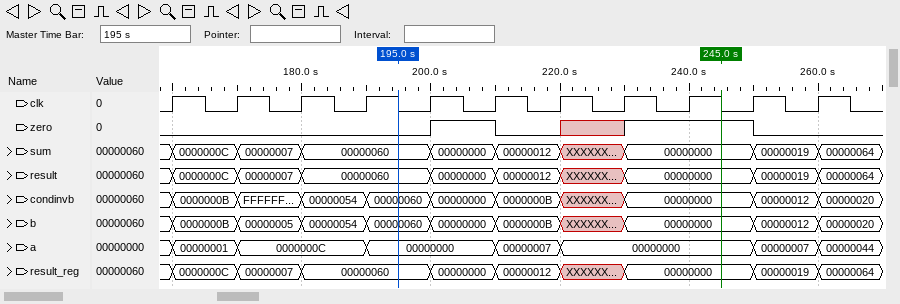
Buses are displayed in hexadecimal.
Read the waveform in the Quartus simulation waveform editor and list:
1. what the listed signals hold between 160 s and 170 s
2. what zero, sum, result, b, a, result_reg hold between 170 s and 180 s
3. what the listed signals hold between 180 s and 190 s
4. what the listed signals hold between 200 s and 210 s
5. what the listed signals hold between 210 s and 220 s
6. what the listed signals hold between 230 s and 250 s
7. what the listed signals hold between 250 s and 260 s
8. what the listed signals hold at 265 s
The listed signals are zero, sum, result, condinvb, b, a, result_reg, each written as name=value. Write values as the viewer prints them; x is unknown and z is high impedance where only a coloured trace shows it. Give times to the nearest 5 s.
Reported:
zero=0, sum=0000000C, result=0000000C, condinvb=0000000B, b=0000000B, a=00000001, result_reg=0000000C
zero=0, sum=00000007, result=00000007, b=00000005, a=0000000C, result_reg=00000007
zero=0, sum=00000060, result=00000060, condinvb=00000054, b=00000054, a=0000000C, result_reg=00000060
zero=1, sum=00000000, result=00000000, condinvb=00000000, b=00000000, a=00000000, result_reg=00000000
zero=0, sum=00000012, result=00000012, condinvb=0000000B, b=0000000B, a=00000007, result_reg=00000012
zero=1, sum=00000000, result=00000000, condinvb=00000000, b=00000000, a=00000000, result_reg=00000000
zero=0, sum=00000019, result=00000019, condinvb=00000012, b=00000012, a=00000007, result_reg=00000019
zero=0, sum=00000064, result=00000064, condinvb=00000020, b=00000020, a=00000044, result_reg=00000064
